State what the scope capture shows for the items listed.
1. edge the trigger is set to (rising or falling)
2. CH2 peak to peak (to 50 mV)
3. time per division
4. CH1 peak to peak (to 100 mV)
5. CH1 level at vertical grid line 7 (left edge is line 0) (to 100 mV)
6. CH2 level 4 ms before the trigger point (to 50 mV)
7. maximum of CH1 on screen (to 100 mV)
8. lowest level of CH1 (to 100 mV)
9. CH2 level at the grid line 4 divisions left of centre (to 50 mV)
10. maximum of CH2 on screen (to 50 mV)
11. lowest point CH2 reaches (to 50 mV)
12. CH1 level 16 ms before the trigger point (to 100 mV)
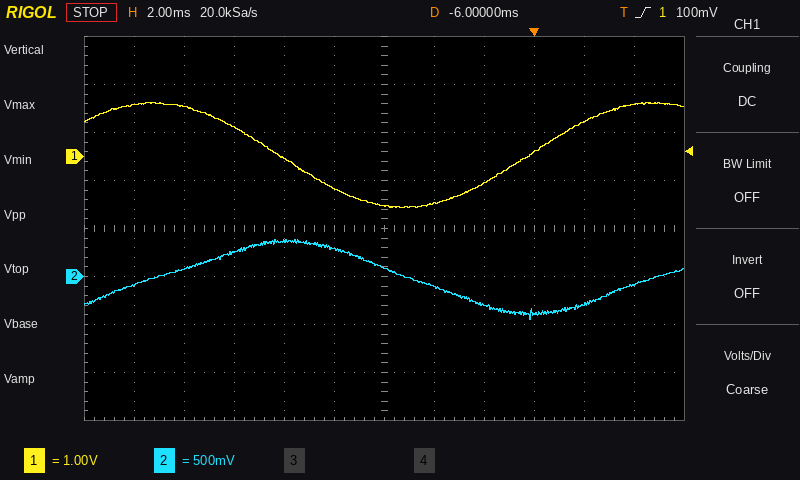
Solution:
rising
850 mV
2 ms
2.2 V
-1.0 V
-100 mV
1.1 V
-1.1 V
100 mV
400 mV
-450 mV
1.1 V
